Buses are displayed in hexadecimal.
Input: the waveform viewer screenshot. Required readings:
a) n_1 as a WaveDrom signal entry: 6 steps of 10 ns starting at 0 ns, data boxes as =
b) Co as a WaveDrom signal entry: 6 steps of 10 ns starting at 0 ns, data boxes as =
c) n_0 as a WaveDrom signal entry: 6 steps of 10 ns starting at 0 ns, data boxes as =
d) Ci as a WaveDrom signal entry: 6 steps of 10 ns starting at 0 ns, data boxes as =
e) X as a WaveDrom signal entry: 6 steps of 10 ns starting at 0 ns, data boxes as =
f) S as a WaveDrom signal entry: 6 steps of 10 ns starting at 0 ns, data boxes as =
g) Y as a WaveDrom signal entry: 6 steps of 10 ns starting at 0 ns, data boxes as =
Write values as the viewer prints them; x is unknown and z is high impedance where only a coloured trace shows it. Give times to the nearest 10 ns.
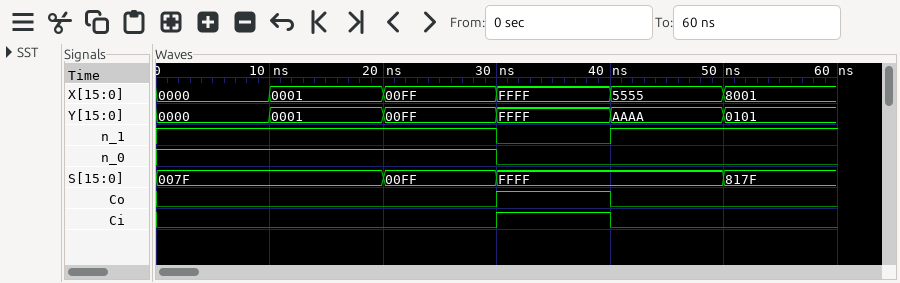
{name: 'n_1', wave: '1..01.'}
{name: 'Co', wave: '0..10.'}
{name: 'n_0', wave: '1..0..'}
{name: 'Ci', wave: '0..10.'}
{name: 'X', wave: '======', data: '0000 0001 00FF FFFF 5555 8001'}
{name: 'S', wave: '=.==.=', data: '007F 00FF FFFF 817F'}
{name: 'Y', wave: '======', data: '0000 0001 00FF FFFF AAAA 0101'}
